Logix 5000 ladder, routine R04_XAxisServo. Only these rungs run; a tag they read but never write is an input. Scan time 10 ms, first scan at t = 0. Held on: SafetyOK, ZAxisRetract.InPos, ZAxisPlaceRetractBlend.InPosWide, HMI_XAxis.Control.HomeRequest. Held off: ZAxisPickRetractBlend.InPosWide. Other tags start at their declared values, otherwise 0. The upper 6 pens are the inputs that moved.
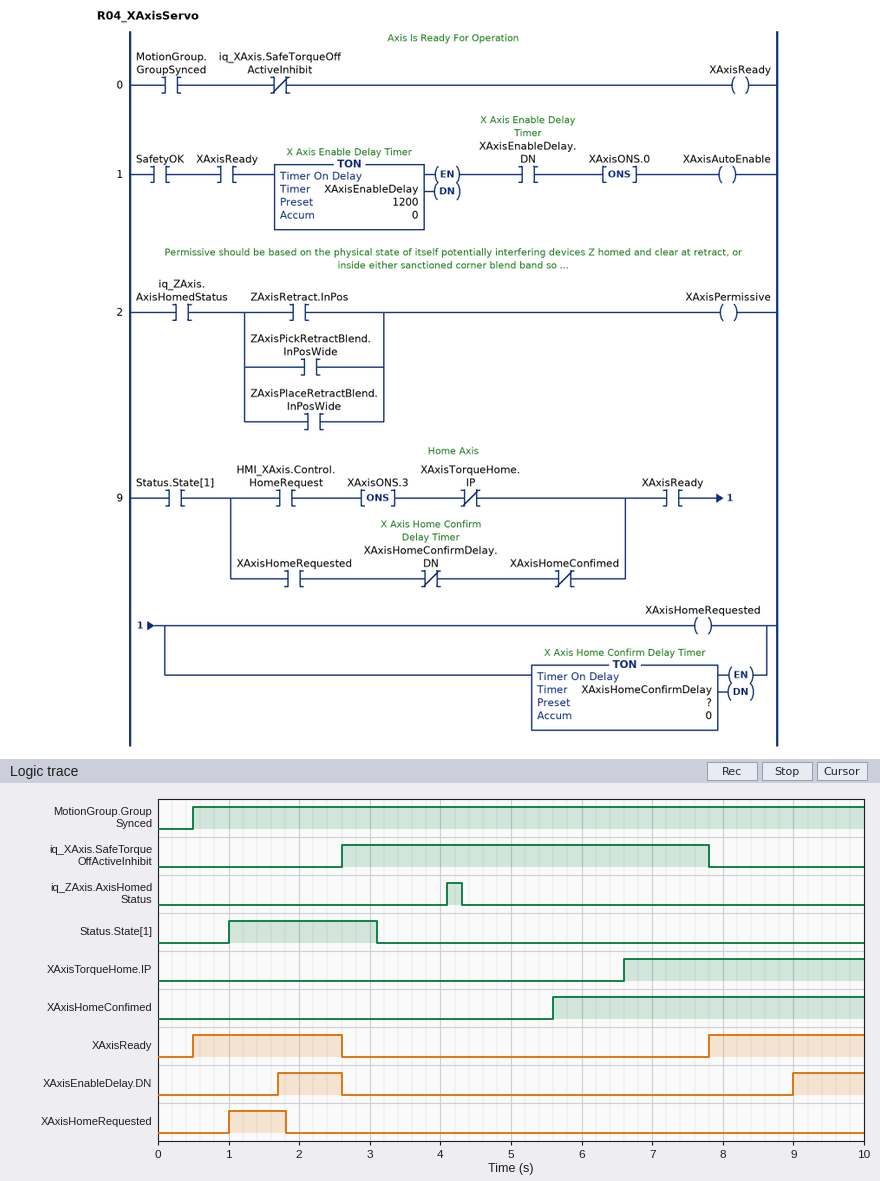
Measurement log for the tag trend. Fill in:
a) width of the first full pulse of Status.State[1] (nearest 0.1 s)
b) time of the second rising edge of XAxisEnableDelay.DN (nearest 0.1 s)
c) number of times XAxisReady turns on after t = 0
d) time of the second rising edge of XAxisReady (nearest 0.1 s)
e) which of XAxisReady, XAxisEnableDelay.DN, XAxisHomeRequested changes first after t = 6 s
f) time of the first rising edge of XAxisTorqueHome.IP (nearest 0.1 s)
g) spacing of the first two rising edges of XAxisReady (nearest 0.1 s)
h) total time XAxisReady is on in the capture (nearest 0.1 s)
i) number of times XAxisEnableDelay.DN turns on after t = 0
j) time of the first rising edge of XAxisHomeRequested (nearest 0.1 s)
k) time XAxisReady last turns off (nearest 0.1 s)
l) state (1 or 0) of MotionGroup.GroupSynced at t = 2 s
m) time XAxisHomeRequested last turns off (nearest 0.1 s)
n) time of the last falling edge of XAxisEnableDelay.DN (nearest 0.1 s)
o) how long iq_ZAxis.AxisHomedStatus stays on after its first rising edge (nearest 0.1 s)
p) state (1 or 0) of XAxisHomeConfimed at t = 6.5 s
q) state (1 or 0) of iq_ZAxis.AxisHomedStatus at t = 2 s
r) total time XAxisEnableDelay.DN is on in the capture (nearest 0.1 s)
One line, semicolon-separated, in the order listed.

2.1 s; 9.0 s; 2; 7.8 s; XAxisReady; 6.6 s; 7.3 s; 4.3 s; 2; 1.0 s; 2.6 s; 1; 1.8 s; 2.6 s; 0.2 s; 1; 0; 1.9 s
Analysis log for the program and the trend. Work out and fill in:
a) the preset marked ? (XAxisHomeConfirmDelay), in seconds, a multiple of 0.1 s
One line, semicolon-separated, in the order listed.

0.8 s
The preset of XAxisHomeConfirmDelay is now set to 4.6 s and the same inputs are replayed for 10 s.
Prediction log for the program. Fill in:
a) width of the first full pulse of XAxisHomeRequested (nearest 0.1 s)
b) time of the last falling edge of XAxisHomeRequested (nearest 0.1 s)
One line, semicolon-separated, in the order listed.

1.6 s; 2.6 s
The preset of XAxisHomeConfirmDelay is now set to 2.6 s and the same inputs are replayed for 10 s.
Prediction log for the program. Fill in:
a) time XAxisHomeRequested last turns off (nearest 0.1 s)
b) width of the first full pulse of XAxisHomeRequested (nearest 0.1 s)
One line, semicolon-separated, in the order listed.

2.6 s; 1.6 s
